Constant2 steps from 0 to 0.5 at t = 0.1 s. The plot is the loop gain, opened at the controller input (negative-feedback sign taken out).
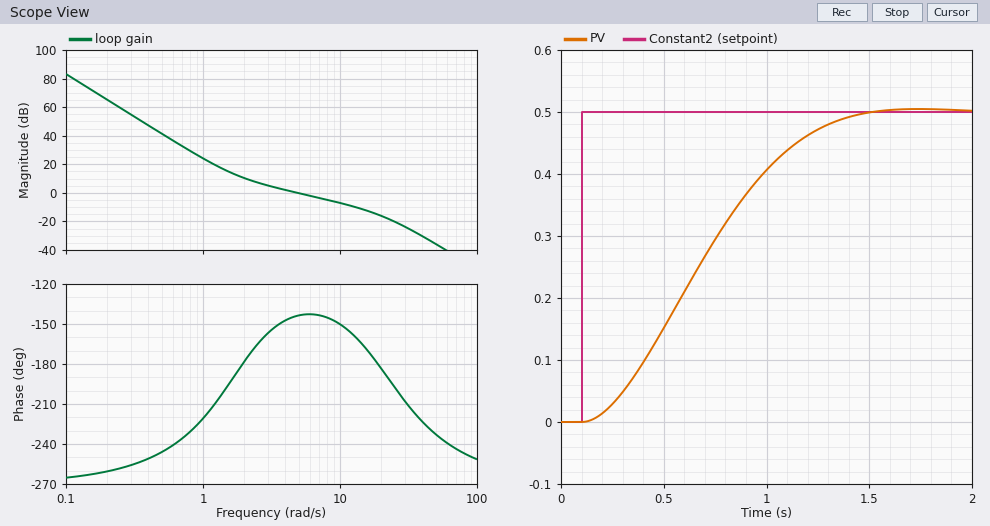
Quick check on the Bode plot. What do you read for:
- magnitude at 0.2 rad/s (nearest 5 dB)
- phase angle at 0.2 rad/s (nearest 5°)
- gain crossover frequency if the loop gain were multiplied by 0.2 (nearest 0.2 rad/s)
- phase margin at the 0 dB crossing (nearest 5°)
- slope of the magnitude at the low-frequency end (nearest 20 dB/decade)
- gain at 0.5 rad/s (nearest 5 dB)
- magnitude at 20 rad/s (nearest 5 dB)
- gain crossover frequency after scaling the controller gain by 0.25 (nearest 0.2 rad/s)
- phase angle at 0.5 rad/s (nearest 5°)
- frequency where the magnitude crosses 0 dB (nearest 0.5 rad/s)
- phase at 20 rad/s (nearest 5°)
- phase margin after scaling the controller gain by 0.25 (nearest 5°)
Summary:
65 dB
-260°
1.6 rad/s
35°
-60 dB/decade
40 dB
-15 dB
1.8 rad/s
-245°
5.0 rad/s
-185°
-5°
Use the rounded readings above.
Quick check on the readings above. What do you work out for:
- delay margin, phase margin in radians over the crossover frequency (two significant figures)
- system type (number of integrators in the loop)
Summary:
0.12 s
3
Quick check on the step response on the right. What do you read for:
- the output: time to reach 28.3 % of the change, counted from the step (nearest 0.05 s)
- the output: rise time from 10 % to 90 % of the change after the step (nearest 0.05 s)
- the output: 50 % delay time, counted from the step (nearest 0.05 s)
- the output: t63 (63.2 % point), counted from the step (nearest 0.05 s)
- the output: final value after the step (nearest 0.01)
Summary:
0.40 s
0.85 s
0.55 s
0.70 s
0.50
